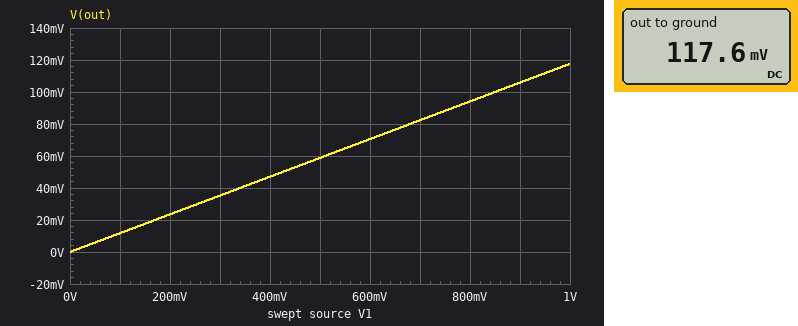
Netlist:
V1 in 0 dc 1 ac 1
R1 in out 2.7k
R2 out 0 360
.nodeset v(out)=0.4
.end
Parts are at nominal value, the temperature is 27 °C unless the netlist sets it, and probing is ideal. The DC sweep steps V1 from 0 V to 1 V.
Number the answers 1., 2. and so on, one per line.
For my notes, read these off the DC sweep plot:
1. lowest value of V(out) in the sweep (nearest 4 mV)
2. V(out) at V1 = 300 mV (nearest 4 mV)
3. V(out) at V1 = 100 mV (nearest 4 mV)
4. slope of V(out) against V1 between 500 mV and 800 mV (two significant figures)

1. 0 V
2. 36 mV
3. 12 mV
4. 0.12 V/V
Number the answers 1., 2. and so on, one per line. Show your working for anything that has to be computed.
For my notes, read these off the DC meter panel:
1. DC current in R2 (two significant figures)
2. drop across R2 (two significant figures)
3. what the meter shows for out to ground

1. (117.6 mV) / 360 Ω = 330 µA
2. 117.6 mV = 120 mV
3. 117.6 mV
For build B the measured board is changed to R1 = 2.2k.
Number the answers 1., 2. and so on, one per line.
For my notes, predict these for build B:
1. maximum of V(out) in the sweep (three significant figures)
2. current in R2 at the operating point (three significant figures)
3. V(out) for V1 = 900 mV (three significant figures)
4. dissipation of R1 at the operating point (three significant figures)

1. 141 mV
2. 391 µA
3. 127 mV
4. 336 µW
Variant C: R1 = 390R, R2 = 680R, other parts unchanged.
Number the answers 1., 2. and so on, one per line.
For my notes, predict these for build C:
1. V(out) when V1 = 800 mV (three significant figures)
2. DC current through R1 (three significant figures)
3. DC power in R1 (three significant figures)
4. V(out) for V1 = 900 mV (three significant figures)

1. 508 mV
2. 935 µA
3. 341 µW
4. 572 mV
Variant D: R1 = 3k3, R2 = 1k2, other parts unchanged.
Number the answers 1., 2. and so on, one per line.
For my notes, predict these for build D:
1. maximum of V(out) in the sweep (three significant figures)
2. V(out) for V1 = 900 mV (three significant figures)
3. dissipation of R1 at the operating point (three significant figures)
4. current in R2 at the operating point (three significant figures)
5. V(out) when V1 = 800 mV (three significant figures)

1. 267 mV
2. 240 mV
3. 163 µW
4. 222 µA
5. 213 mV
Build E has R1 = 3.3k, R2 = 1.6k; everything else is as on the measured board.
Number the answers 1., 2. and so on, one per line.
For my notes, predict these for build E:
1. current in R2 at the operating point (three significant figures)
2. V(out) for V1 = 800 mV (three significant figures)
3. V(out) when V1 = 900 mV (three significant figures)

1. 204 µA
2. 261 mV
3. 294 mV
